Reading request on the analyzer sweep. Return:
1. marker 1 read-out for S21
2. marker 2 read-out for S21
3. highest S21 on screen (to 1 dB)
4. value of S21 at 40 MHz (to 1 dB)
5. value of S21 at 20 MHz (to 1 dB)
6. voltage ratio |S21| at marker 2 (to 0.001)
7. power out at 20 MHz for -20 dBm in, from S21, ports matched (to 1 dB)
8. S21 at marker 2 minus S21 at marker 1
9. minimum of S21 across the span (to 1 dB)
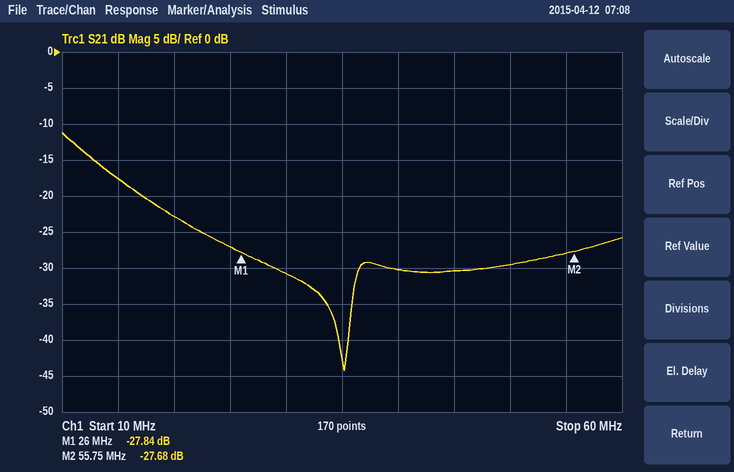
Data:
-27.84 dB
-27.68 dB
-11 dB
-30 dB
-23 dB
0.041
-43 dBm
0.16 dB
-44 dB
